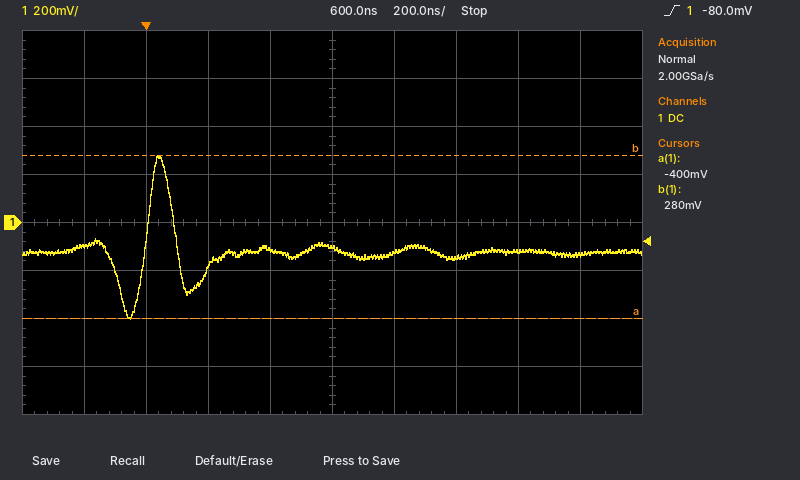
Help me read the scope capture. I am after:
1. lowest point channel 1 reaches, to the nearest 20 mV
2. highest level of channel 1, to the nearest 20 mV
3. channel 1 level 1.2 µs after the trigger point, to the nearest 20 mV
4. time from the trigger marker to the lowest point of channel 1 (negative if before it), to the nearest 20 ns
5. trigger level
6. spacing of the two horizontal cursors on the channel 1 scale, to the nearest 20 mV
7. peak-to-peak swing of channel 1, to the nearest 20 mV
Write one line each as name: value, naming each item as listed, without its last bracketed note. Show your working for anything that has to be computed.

lowest point channel 1 reaches, to the nearest 20 mV: -400 mV
highest level of channel 1, to the nearest 20 mV: 280 mV
channel 1 level 1.2 µs after the trigger point, to the nearest 20 mV: -120 mV
time from the trigger marker to the lowest point of channel 1 (negative if before it), to the nearest 20 ns: -60 ns
trigger level: -80.0 mV
spacing of the two horizontal cursors on the channel 1 scale, to the nearest 20 mV: 680 mV
peak-to-peak swing of channel 1, to the nearest 20 mV: 280 mV − (-400 mV) = 680 mV
